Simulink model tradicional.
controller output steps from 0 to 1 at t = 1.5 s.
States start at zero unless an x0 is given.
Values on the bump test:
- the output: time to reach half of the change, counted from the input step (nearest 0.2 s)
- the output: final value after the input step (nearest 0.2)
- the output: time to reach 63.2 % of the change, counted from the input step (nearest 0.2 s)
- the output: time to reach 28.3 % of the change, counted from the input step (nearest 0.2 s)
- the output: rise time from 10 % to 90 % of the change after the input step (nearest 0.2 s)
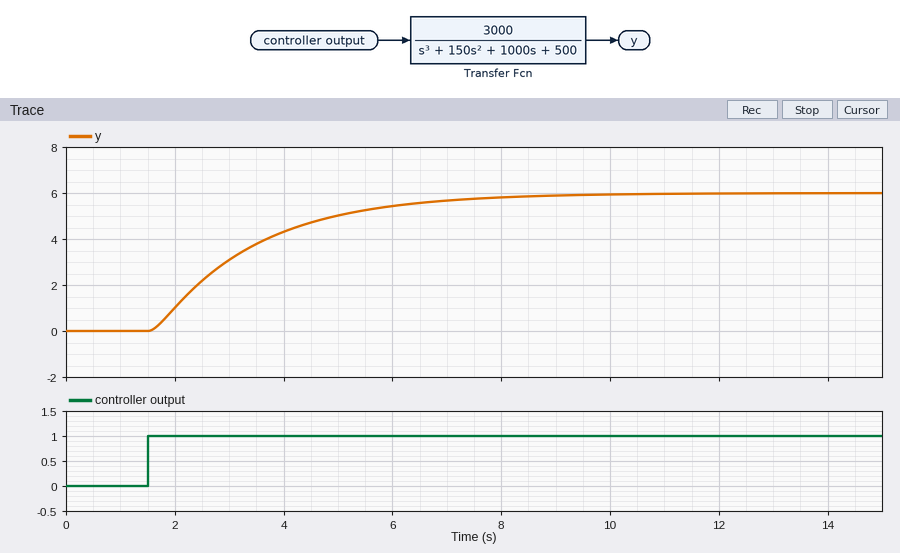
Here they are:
1.4 s
6.0
2.0 s
0.8 s
4.0 s
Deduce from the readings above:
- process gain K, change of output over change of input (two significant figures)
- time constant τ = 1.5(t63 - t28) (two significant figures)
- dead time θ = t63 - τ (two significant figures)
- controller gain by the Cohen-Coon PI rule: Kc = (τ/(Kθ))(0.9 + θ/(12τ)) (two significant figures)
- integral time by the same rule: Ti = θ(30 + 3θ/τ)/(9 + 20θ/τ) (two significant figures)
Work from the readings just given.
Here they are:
6.0
1.8 s
0.20 s
1.4
0.54 s
